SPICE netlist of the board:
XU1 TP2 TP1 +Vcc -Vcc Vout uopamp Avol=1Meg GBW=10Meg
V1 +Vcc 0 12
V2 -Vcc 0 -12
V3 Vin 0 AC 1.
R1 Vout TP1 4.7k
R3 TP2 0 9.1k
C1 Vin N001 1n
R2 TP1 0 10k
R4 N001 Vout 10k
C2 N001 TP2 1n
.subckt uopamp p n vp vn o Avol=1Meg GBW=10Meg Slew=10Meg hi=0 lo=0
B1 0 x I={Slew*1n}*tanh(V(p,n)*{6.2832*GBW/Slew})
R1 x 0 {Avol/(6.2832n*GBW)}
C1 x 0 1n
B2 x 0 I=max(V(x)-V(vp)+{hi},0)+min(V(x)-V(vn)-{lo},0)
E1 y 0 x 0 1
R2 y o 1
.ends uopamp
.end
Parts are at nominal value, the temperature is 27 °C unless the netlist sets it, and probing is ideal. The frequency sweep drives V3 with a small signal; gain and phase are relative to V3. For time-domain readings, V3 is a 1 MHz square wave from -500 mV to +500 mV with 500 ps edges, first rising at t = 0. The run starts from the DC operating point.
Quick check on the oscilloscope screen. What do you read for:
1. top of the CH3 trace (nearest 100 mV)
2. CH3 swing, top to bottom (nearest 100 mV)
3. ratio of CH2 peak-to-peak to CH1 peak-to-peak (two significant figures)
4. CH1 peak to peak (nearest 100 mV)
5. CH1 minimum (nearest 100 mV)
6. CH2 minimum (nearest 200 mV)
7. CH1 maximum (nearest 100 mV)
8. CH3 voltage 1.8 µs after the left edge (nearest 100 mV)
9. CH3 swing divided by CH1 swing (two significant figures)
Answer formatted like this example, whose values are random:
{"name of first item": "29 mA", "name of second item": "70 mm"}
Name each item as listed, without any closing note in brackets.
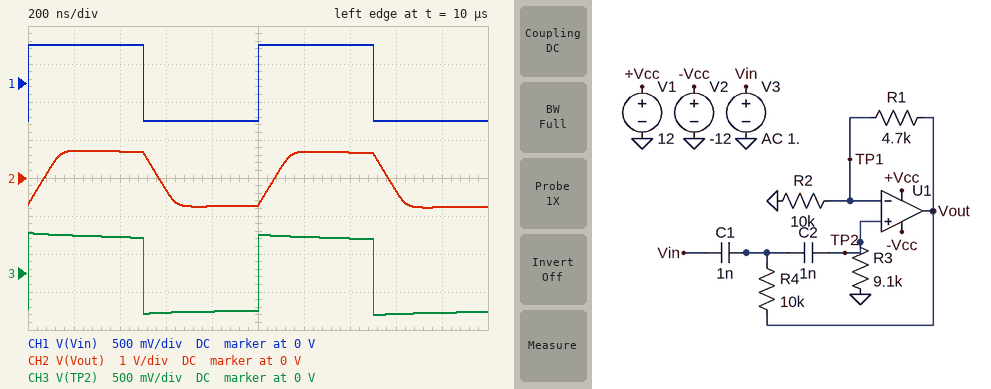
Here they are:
{"top of the CH3 trace": "500 mV", "CH3 swing, top to bottom": "1.1 V", "ratio of CH2 peak-to-peak to CH1 peak-to-peak": "1.5", "CH1 peak to peak": "1.0 V", "CH1 minimum": "-500 mV", "CH2 minimum": "-800 mV", "CH1 maximum": "500 mV", "CH3 voltage 1.8 µs after the left edge": "-500 mV", "CH3 swing divided by CH1 swing": "1.1"}
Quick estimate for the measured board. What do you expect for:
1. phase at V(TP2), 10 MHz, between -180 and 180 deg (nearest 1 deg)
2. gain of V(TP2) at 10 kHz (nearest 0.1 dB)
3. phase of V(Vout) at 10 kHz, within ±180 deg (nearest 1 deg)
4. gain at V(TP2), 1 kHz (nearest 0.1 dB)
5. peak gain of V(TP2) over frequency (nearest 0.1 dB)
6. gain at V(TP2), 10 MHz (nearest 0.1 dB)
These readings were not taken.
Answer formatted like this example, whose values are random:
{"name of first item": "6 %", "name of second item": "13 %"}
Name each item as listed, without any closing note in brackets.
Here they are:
{"phase at V(TP2), 10 MHz, between -180 and 180 deg": "0 deg", "gain of V(TP2) at 10 kHz": "-10.3 dB", "phase of V(Vout) at 10 kHz, within ±180 deg": "123 deg", "gain at V(TP2), 1 kHz": "-48.9 dB", "peak gain of V(TP2) over frequency": "0 dB", "gain at V(TP2), 10 MHz": "0 dB"}
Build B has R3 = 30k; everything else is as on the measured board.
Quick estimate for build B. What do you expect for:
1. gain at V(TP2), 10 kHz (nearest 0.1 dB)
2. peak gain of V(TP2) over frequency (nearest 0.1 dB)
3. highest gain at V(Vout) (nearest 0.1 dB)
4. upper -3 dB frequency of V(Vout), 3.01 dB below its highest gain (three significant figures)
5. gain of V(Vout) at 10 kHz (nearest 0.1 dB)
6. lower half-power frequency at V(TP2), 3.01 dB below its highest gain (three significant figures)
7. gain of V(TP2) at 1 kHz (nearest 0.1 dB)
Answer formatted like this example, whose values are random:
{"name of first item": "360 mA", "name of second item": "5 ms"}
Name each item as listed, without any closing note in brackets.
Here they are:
{"gain at V(TP2), 10 kHz": "9.1 dB", "peak gain of V(TP2) over frequency": "9.5 dB", "highest gain at V(Vout)": "12.8 dB", "upper -3 dB frequency of V(Vout), 3.01 dB below its highest gain": "11.8 kHz", "gain of V(Vout) at 10 kHz": "12.4 dB", "lower half-power frequency at V(TP2), 3.01 dB below its highest gain": "8.12 kHz", "gain of V(TP2) at 1 kHz": "-38.4 dB"}
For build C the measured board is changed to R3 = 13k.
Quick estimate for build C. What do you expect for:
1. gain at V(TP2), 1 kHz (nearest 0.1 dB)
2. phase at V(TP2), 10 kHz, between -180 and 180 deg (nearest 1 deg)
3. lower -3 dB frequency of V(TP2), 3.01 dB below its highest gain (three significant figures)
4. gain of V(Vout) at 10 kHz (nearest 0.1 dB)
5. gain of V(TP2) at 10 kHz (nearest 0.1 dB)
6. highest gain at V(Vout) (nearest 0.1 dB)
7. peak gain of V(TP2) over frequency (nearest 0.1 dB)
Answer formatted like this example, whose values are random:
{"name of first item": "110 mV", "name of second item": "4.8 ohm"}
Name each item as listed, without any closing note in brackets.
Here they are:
{"gain at V(TP2), 1 kHz": "-45.8 dB", "phase at V(TP2), 10 kHz, between -180 and 180 deg": "119 deg", "lower -3 dB frequency of V(TP2), 3.01 dB below its highest gain": "12.6 kHz", "gain of V(Vout) at 10 kHz": "-2.4 dB", "gain of V(TP2) at 10 kHz": "-5.8 dB", "highest gain at V(Vout)": "3.6 dB", "peak gain of V(TP2) over frequency": "0.3 dB"}
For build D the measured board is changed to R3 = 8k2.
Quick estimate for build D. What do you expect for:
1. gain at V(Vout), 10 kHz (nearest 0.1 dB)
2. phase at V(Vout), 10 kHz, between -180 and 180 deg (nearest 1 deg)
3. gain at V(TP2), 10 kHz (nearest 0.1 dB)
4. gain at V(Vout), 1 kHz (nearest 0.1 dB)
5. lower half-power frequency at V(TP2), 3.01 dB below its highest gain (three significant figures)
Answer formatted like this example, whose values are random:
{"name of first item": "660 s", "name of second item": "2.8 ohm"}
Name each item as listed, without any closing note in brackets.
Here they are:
{"gain at V(Vout), 10 kHz": "-8.2 dB", "phase at V(Vout), 10 kHz, between -180 and 180 deg": "124 deg", "gain at V(TP2), 10 kHz": "-11.5 dB", "gain at V(Vout), 1 kHz": "-46.5 dB", "lower half-power frequency at V(TP2), 3.01 dB below its highest gain": "23.3 kHz"}
